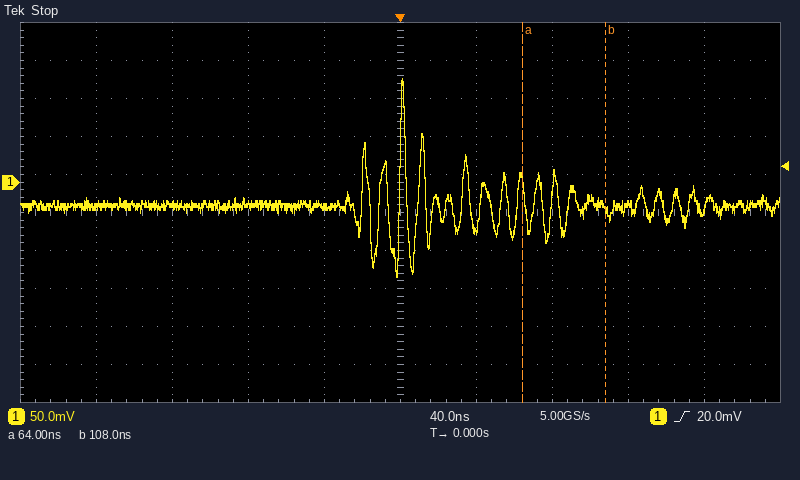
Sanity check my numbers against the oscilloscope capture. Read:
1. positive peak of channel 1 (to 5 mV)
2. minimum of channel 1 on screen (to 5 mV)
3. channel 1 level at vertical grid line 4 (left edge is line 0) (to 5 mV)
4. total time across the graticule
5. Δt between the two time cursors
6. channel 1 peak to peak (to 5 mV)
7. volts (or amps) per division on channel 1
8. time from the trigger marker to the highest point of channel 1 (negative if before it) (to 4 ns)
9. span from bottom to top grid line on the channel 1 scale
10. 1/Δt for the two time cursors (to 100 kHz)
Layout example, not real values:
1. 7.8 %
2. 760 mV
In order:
1. 135 mV
2. -125 mV
3. -30 mV
4. 400 ns
5. 44 ns
6. 260 mV
7. 50 mV
8. 0 ns
9. 500 mV
10. 22.7 MHz
